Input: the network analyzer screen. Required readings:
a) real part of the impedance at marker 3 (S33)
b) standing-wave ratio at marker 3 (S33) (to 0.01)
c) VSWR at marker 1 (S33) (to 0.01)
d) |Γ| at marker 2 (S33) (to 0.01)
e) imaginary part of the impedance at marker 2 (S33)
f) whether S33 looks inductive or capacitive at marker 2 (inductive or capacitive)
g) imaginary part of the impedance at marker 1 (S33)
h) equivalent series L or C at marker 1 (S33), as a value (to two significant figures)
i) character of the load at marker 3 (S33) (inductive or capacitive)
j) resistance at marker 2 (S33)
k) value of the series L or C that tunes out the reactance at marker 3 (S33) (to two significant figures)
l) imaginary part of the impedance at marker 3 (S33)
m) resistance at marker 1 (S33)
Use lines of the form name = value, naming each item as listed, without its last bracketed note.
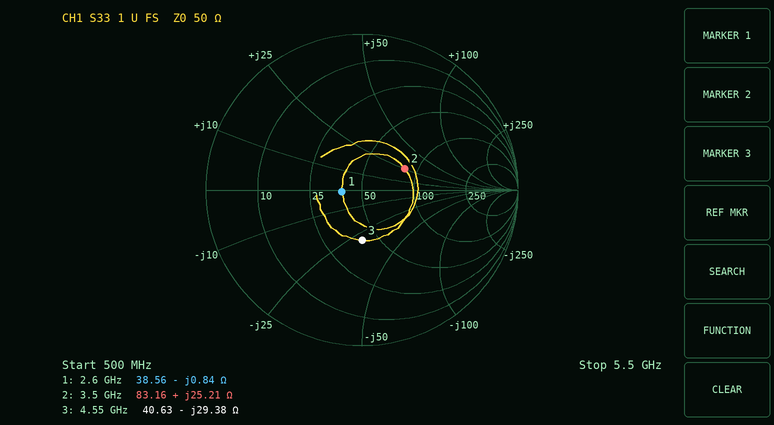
real part of the impedance at marker 3 = 40.63 Ω
standing-wave ratio at marker 3 (S33) = 1.96
VSWR at marker 1 (S33) = 1.30
|Γ| at marker 2 (S33) = 0.31
imaginary part of the impedance at marker 2 = +25.21 Ω
whether S33 looks inductive or capacitive at marker 2 = inductive
imaginary part of the impedance at marker 1 = -0.84 Ω
equivalent series L or C at marker 1 (S33), as a value = 73 pF
character of the load at marker 3 (S33) = capacitive
resistance at marker 2 = 83.16 Ω
value of the series L or C that tunes out the reactance at marker 3 (S33) = 1.0 nH
imaginary part of the impedance at marker 3 = -29.38 Ω
resistance at marker 1 = 38.56 Ω
